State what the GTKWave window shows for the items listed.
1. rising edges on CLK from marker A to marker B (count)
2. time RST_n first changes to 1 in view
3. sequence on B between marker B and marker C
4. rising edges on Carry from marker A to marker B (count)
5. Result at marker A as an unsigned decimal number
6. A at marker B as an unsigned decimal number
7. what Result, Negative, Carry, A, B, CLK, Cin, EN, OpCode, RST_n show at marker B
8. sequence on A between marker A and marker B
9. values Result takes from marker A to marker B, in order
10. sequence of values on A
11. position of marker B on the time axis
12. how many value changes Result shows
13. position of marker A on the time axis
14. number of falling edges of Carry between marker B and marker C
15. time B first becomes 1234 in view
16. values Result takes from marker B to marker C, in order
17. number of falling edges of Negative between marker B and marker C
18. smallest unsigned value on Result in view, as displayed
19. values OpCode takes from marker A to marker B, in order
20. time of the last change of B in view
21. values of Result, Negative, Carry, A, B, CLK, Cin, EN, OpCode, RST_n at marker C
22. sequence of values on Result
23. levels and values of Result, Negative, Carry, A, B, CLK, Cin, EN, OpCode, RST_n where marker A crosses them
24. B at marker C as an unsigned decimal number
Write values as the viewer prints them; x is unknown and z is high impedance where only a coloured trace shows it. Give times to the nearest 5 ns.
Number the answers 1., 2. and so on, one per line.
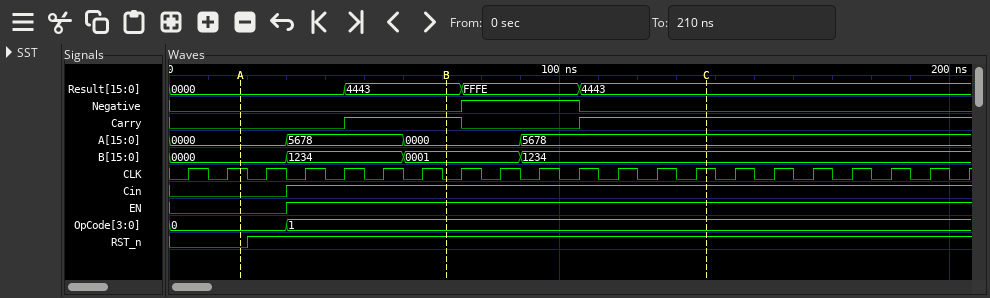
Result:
1. 5
2. 20 ns
3. 0001, 1234
4. 1
5. 0
6. 0
7. Result=4443, Negative=0, Carry=1, A=0000, B=0001, CLK=0, Cin=1, EN=1, OpCode=1, RST_n=1
8. 0000, 5678, 0000
9. 0000, 4443
10. 0000, 5678, 0000, 5678
11. 70 ns
12. 3
13. 20 ns
14. 1
15. 30 ns
16. 4443, FFFE, 4443
17. 1
18. 0000
19. 0, 1
20. 90 ns
21. Result=4443, Negative=0, Carry=1, A=5678, B=1234, CLK=1, Cin=1, EN=1, OpCode=1, RST_n=1
22. 0000, 4443, FFFE, 4443
23. Result=0000, Negative=0, Carry=0, A=0000, B=0000, CLK=1, Cin=0, EN=0, OpCode=0, RST_n=0
24. 4660
